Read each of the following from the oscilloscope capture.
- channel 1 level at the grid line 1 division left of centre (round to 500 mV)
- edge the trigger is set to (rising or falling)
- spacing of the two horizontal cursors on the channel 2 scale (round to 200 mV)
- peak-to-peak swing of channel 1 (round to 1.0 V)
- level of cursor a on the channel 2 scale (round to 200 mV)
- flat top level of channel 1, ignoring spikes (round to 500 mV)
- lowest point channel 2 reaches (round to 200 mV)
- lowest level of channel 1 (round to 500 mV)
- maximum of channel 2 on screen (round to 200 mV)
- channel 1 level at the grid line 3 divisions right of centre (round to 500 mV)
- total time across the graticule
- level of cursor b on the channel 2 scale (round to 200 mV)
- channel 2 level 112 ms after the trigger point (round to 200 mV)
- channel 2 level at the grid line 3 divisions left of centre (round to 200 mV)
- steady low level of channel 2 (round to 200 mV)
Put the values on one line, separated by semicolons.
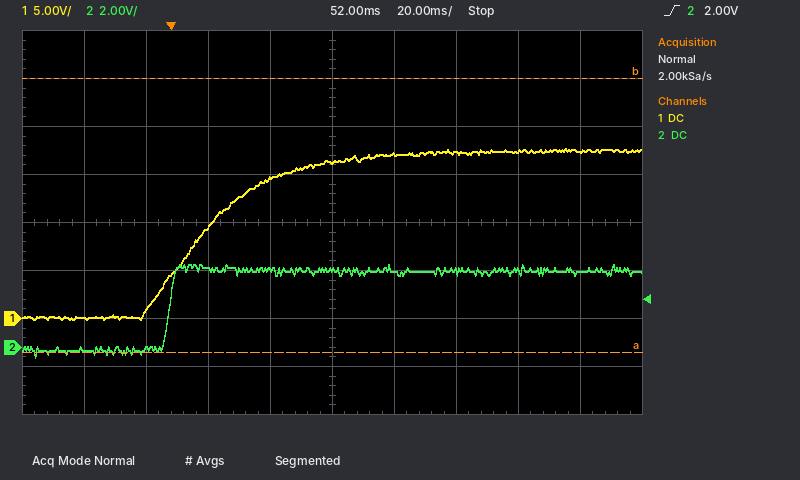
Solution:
14.5 V; rising; 11.4 V; 18.0 V; -200 mV; 17.5 V; -400 mV; 0.0 V; 3.4 V; 17.5 V; 200 ms; 11.2 V; 3.2 V; 0.0 V; -200 mV
